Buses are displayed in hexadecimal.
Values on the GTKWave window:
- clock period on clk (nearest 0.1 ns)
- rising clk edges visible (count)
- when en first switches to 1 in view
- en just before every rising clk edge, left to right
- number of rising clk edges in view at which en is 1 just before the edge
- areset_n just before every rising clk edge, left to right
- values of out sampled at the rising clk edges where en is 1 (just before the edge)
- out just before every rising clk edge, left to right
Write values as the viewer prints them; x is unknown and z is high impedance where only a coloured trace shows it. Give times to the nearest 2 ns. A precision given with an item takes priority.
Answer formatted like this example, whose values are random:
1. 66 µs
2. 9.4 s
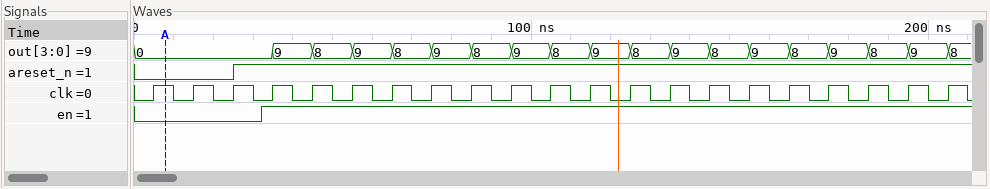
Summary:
1. 10 ns
2. 21
3. 32 ns
4. 0 0 0 1 1 1 1 1 1 1 1 1 1 1 1 1 1 1 1 1 1
5. 18
6. 0 0 0 1 1 1 1 1 1 1 1 1 1 1 1 1 1 1 1 1 1
7. 0, 9, 8, 9, 8, 9, 8, 9, 8, 9, 8, 9, 8, 9, 8, 9, 8, 9
8. 0, 0, 0, 0, 9, 8, 9, 8, 9, 8, 9, 8, 9, 8, 9, 8, 9, 8, 9, 8, 9
